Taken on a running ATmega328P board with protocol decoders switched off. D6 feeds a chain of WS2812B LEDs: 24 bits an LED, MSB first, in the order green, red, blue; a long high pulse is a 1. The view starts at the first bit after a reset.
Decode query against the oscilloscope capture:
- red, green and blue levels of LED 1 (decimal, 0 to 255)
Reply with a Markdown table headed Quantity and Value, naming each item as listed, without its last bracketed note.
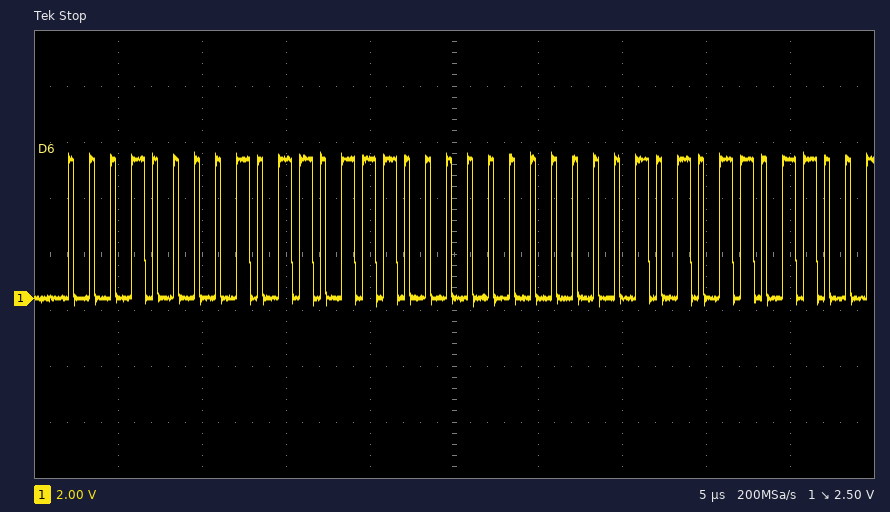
| Quantity | Value |
|---|---|
| red, green and blue levels of LED 1 | 183, 16, 0 |
